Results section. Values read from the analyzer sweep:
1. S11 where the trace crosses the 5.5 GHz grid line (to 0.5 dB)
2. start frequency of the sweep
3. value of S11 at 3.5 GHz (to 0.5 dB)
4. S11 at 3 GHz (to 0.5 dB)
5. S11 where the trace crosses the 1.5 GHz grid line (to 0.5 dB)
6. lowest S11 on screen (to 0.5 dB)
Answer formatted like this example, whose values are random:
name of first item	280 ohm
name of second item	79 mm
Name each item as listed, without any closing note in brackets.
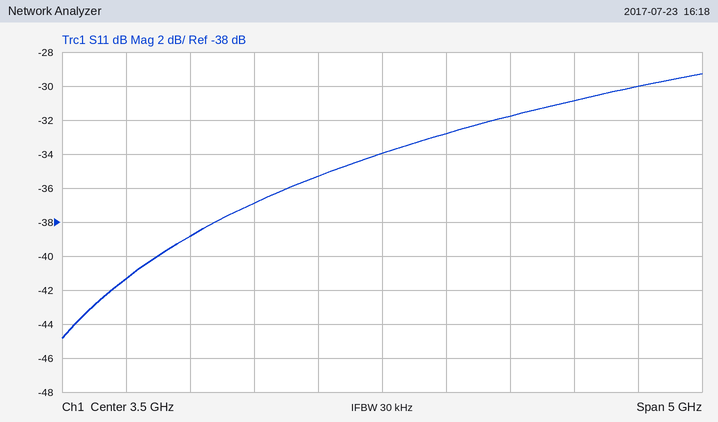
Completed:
S11 where the trace crosses the 5.5 GHz grid line	-30.0 dB
start frequency of the sweep	1 GHz
value of S11 at 3.5 GHz	-34.0 dB
S11 at 3 GHz	-35.5 dB
S11 where the trace crosses the 1.5 GHz grid line	-41.5 dB
lowest S11 on screen	-45.0 dB
